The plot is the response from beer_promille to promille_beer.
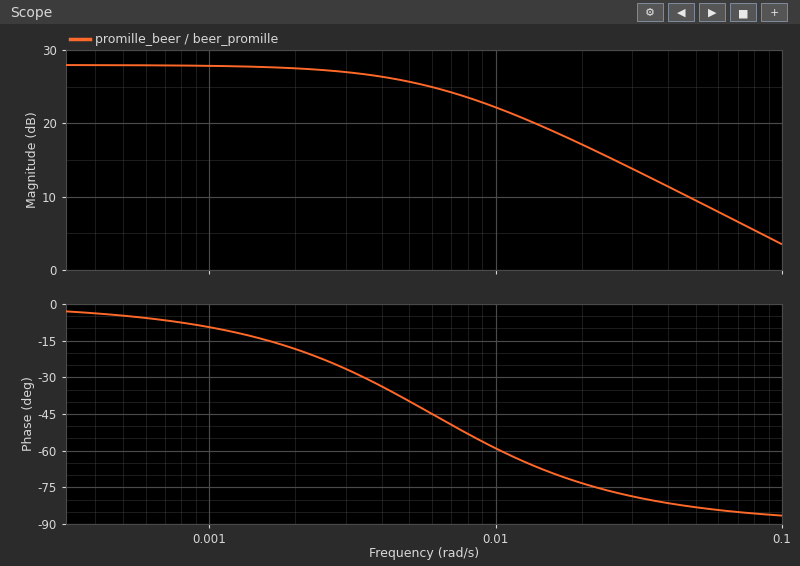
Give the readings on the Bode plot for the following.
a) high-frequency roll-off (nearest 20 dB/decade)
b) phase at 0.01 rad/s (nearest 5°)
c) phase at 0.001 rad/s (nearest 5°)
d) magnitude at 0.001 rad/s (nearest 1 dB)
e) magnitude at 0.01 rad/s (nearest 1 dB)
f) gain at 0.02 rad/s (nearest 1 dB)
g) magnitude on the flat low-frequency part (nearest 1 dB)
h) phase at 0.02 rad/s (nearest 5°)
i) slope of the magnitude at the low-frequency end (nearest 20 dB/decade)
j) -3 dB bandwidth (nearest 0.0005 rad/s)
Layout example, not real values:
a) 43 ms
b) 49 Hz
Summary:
a) -20 dB/decade
b) -60°
c) -10°
d) 28 dB
e) 22 dB
f) 17 dB
g) 28 dB
h) -75°
i) 0 dB/decade
j) 0.0060 rad/s
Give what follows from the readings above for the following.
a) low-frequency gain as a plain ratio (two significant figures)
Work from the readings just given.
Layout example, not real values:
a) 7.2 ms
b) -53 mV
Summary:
a) 25
